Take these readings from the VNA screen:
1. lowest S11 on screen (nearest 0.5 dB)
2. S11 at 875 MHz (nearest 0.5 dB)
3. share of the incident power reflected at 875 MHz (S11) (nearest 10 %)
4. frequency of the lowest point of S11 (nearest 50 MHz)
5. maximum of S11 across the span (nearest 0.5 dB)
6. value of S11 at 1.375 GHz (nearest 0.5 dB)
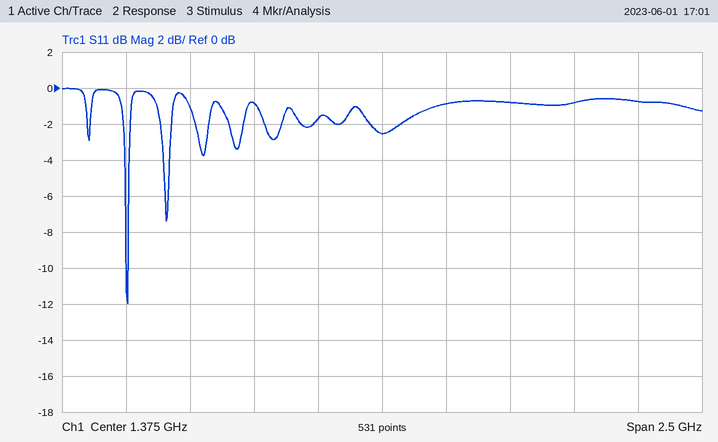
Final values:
-12.0 dB
-1.0 dB
80 %
400 MHz
0.0 dB
-2.5 dB
